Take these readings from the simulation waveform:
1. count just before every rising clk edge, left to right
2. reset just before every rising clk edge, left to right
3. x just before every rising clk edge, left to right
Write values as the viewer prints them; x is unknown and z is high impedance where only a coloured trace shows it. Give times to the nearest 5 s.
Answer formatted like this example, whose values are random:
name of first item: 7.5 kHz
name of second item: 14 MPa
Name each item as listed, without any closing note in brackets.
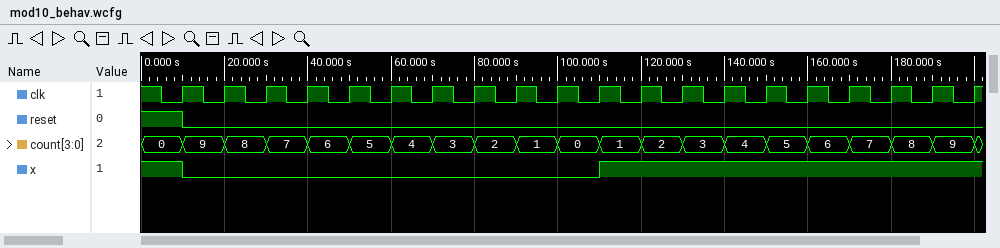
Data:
count just before every rising clk edge, left to right: 0, 9, 8, 7, 6, 5, 4, 3, 2, 1, 0, 1, 2, 3, 4, 5, 6, 7, 8, 9
reset just before every rising clk edge, left to right: 1 0 0 0 0 0 0 0 0 0 0 0 0 0 0 0 0 0 0 0
x just before every rising clk edge, left to right: 1 0 0 0 0 0 0 0 0 0 0 1 1 1 1 1 1 1 1 1
